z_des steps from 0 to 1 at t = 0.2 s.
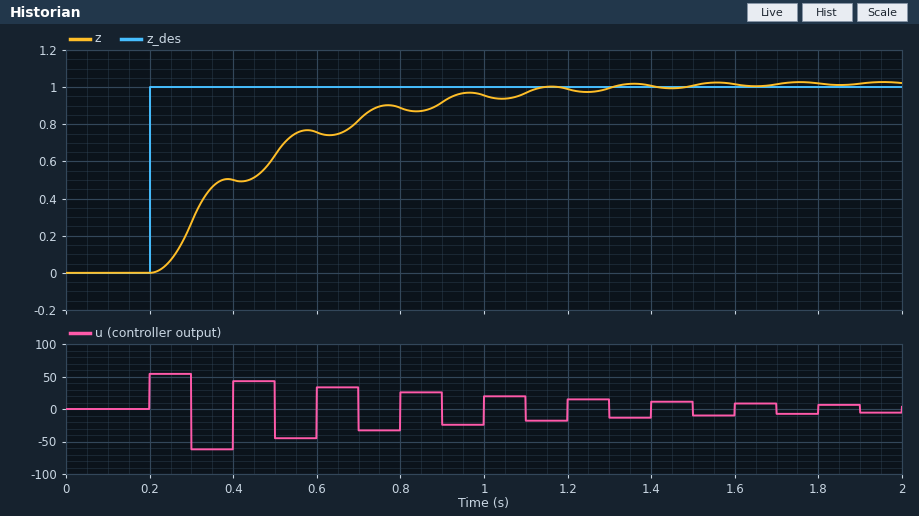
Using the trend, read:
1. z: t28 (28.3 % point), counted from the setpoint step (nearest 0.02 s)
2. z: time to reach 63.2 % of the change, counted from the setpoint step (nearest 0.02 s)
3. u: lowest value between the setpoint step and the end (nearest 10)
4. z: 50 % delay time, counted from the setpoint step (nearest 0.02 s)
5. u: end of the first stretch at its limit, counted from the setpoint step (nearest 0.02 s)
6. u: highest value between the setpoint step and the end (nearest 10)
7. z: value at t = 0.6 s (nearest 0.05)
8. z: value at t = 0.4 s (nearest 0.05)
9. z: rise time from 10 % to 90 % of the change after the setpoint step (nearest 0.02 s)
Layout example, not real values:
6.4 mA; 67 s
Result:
0.10 s; 0.30 s; -60; 0.24 s; 0.10 s; 50; 0.75; 0.50; 0.64 s
